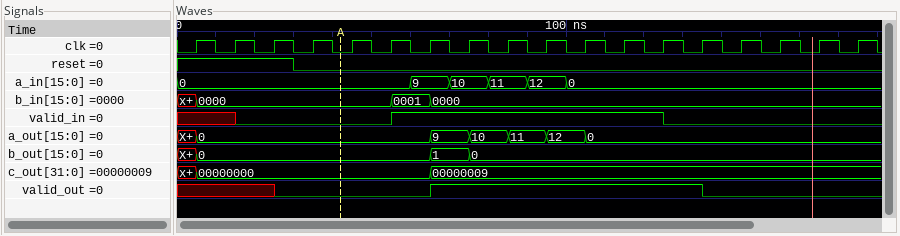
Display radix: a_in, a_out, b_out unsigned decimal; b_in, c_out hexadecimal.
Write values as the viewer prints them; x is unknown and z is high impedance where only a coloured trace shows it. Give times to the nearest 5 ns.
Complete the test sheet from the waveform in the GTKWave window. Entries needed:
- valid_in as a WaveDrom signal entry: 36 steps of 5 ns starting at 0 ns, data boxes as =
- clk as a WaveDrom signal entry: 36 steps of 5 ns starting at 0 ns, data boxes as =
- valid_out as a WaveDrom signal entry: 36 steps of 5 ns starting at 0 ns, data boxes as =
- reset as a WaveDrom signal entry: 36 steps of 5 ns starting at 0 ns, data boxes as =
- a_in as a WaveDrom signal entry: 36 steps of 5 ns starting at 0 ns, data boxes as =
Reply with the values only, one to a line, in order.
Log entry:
{name: 'valid_in', wave: 'x..0.......1.............0..........'}
{name: 'clk', wave: '010101010101010101010101010101010101'}
{name: 'valid_out', wave: 'x....0.......1.............0........'}
{name: 'reset', wave: '1.....0.............................'}
{name: 'a_in', wave: '=...........=.=.=.=.=...............', data: '0 9 10 11 12 0'}
